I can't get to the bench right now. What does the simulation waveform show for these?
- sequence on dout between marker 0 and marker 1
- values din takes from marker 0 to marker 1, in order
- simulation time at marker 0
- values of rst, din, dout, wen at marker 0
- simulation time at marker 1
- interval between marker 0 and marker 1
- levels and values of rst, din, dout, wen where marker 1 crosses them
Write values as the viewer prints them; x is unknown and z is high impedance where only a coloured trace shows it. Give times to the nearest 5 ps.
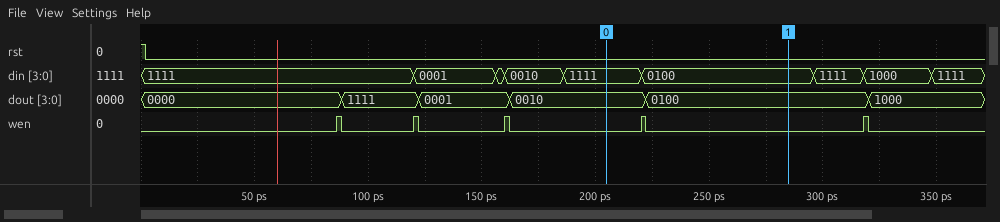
0010, 0100
1111, 0100
205 ps
rst=0, din=1111, dout=0010, wen=0
285 ps
80 ps
rst=0, din=0100, dout=0100, wen=0
